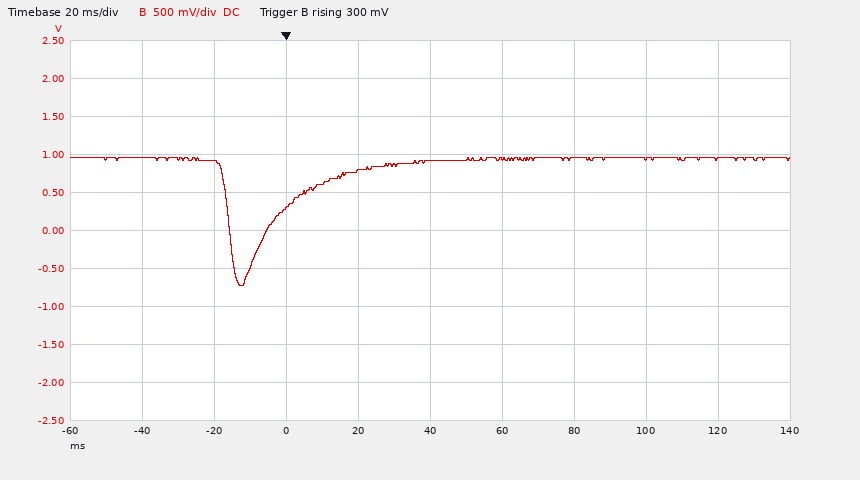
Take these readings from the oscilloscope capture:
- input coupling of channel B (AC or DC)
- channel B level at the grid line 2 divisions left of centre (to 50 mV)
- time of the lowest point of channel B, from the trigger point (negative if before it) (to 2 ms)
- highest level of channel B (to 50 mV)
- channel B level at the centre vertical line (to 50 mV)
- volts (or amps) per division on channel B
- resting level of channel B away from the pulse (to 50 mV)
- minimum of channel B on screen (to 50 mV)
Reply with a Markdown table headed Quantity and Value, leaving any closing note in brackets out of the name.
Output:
| Quantity | Value |
|---|---|
| input coupling of channel B | DC |
| channel B level at the grid line 2 divisions left of centre | 300 mV |
| time of the lowest point of channel B, from the trigger point (negative if before it) | -12 ms |
| highest level of channel B | 950 mV |
| channel B level at the centre vertical line | 900 mV |
| volts (or amps) per division on channel B | 500 mV |
| resting level of channel B away from the pulse | 950 mV |
| minimum of channel B on screen | -700 mV |
